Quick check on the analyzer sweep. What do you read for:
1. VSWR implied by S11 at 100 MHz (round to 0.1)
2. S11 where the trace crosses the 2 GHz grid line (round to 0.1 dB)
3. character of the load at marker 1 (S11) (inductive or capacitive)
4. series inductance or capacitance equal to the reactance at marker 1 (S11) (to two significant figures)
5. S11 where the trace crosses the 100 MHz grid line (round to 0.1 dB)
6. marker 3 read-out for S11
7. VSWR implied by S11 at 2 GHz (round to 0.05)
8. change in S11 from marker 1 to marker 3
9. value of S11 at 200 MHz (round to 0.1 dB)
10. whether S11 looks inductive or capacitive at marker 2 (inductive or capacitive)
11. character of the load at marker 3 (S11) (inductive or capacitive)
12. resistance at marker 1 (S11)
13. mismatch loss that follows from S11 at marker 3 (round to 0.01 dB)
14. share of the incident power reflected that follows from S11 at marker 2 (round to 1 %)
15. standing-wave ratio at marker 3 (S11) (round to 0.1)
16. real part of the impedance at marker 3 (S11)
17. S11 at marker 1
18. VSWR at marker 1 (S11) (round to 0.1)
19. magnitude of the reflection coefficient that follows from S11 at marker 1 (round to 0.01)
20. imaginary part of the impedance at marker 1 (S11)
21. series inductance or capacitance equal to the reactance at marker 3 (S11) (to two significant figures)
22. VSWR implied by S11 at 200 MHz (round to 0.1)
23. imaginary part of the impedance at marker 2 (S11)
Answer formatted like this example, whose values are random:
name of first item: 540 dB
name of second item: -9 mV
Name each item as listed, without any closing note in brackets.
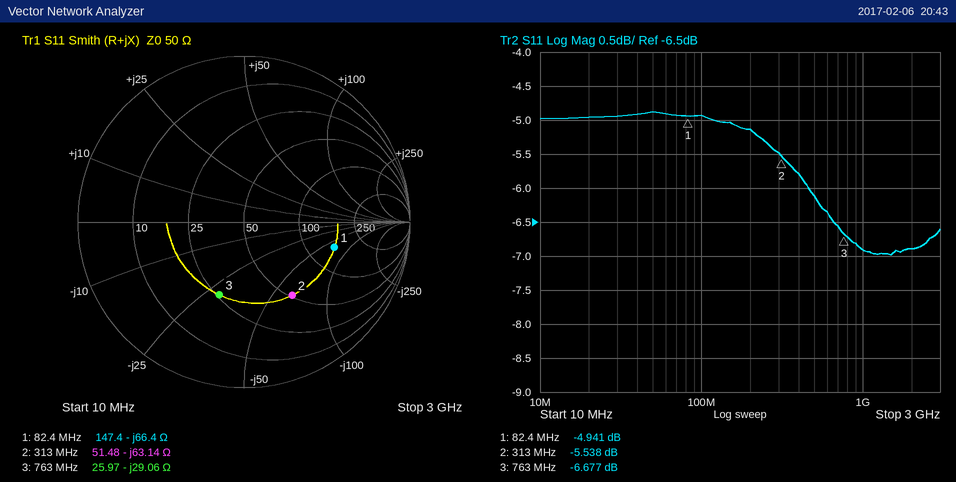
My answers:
VSWR implied by S11 at 100 MHz: 3.6
S11 where the trace crosses the 2 GHz grid line: -6.9 dB
character of the load at marker 1 (S11): capacitive
series inductance or capacitance equal to the reactance at marker 1 (S11): 29 pF
S11 where the trace crosses the 100 MHz grid line: -4.9 dB
marker 3 read-out for S11: -6.677 dB
VSWR implied by S11 at 2 GHz: 2.65
change in S11 from marker 1 to marker 3: -1.736 dB
value of S11 at 200 MHz: -5.1 dB
whether S11 looks inductive or capacitive at marker 2: capacitive
character of the load at marker 3 (S11): capacitive
resistance at marker 1: 147.4 Ω
mismatch loss that follows from S11 at marker 3: 1.05 dB
share of the incident power reflected that follows from S11 at marker 2: 28 %
standing-wave ratio at marker 3 (S11): 2.7
real part of the impedance at marker 3: 25.97 Ω
S11 at marker 1: -4.941 dB
VSWR at marker 1 (S11): 3.6
magnitude of the reflection coefficient that follows from S11 at marker 1: 0.57
imaginary part of the impedance at marker 1: -66.4 Ω
series inductance or capacitance equal to the reactance at marker 3 (S11): 7.2 pF
VSWR implied by S11 at 200 MHz: 3.5
imaginary part of the impedance at marker 2: -63.14 Ω
